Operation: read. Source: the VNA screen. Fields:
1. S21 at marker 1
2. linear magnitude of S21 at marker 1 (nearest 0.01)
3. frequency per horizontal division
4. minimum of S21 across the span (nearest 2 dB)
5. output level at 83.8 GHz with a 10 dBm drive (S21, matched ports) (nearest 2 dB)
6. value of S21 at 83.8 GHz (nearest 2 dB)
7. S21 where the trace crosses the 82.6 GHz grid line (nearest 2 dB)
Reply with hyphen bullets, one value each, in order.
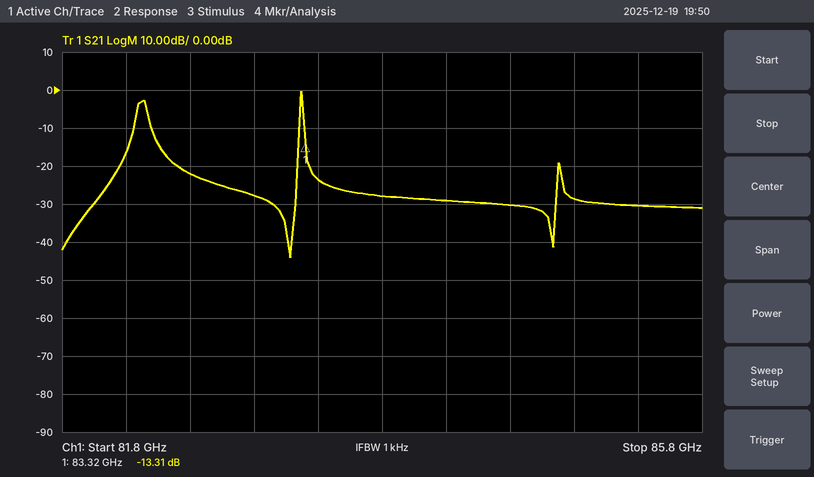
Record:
- -13.31 dB
- 0.22
- 400 MHz
- -44 dB
- -18 dBm
- -28 dB
- -22 dB
